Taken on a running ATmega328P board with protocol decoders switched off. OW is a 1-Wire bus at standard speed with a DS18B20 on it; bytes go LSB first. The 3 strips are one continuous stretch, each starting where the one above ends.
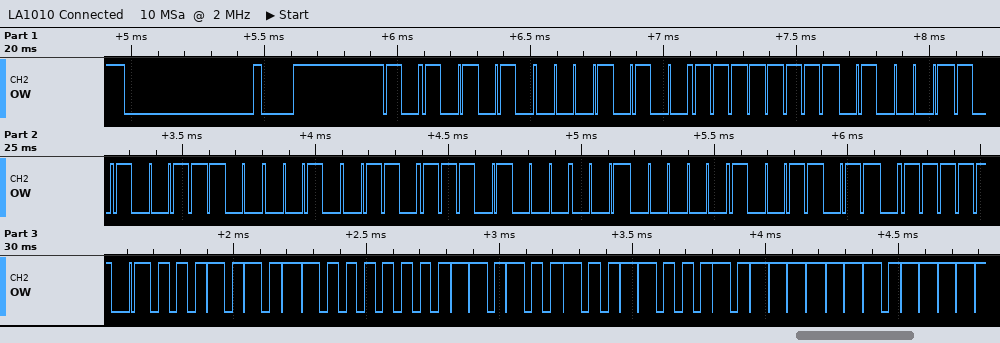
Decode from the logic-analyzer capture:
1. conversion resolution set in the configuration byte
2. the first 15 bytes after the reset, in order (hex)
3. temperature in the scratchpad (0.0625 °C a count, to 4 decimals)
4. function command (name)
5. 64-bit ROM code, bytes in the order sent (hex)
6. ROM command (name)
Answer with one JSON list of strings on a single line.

["12 bits", "55 28 FF 62 39 64 17 04 D9 BE A8 01 4B 46 7F", "26.5000 °C", "Read Scratchpad", "28 FF 62 39 64 17 04 D9", "Match ROM"]
